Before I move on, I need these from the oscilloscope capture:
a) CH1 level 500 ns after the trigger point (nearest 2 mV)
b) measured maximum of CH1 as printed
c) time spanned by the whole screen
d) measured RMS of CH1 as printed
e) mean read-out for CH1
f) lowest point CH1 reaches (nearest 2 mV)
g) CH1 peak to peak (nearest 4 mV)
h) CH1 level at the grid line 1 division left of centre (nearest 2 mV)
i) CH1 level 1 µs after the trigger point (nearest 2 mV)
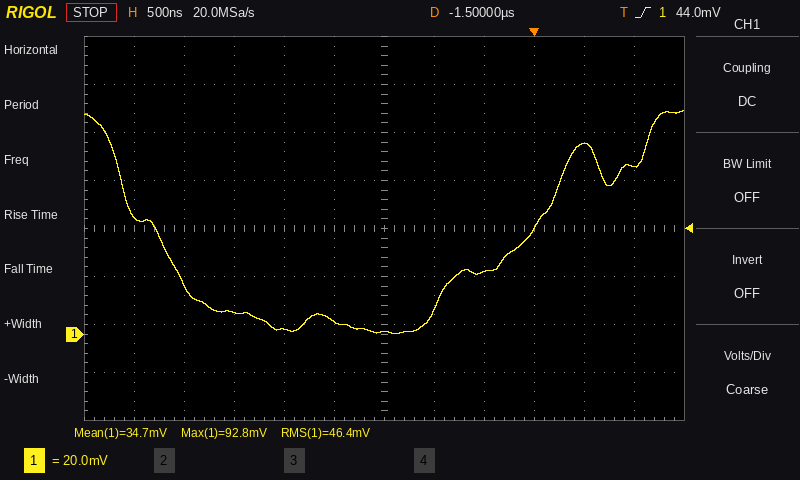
80 mV
92.8 mV
6 µs
46.4 mV
34.7 mV
0 mV
92 mV
6 mV
70 mV
